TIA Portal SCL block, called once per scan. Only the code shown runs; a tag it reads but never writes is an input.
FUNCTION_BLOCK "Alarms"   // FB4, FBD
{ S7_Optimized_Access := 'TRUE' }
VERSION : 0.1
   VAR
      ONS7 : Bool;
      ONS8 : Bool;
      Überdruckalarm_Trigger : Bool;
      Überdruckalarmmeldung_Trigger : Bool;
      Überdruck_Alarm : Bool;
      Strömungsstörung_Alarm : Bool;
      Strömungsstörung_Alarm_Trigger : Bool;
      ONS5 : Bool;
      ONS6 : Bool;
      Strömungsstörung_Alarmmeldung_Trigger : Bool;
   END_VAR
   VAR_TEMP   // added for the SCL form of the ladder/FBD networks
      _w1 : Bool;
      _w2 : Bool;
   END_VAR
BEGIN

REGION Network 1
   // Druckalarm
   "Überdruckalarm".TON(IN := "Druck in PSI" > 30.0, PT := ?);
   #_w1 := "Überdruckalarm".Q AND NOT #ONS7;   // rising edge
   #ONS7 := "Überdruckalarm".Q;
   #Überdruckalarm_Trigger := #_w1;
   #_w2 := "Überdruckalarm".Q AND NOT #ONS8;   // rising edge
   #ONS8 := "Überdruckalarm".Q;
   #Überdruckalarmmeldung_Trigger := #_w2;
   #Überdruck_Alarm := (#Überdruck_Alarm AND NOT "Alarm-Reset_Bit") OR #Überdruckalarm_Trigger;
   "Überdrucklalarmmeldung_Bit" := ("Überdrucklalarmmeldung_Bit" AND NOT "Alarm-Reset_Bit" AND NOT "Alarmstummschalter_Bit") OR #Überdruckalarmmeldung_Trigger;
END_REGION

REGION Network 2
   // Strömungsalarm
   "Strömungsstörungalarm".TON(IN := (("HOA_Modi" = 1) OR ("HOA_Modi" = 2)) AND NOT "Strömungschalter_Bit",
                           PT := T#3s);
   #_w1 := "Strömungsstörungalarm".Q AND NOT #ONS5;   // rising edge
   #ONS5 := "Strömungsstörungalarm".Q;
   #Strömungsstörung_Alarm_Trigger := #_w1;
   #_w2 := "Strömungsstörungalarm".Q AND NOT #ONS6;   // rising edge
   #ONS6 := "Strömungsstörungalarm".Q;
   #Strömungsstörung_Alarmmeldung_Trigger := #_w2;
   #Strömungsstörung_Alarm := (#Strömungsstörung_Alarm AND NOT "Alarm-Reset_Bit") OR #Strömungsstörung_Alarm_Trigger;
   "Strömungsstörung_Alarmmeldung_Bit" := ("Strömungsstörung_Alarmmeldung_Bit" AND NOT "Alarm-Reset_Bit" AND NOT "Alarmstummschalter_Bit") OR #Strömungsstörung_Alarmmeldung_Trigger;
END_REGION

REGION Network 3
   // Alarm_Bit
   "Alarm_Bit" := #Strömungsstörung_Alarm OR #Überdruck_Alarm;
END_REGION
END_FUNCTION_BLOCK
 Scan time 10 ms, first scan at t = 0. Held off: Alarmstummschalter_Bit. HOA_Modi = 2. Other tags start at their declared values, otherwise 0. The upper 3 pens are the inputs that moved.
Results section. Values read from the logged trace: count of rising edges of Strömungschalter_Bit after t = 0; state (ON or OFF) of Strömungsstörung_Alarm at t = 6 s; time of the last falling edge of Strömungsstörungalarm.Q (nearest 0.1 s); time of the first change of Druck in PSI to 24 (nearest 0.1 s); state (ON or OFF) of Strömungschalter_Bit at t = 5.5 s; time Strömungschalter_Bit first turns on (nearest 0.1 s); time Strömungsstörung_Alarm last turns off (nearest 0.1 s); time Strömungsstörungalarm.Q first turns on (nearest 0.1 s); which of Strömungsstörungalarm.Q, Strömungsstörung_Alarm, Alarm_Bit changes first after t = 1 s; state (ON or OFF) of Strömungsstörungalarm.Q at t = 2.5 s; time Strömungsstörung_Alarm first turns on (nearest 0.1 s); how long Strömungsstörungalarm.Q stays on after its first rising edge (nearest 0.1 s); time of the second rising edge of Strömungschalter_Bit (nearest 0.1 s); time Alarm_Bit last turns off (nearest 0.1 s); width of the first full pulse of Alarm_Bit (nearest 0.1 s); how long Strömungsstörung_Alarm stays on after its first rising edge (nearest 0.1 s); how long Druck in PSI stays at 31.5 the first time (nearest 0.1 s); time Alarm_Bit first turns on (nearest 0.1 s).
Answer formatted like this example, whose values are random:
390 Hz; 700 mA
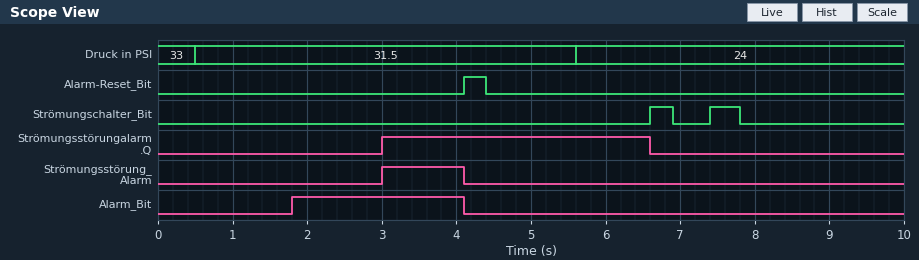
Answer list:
2; OFF; 6.6 s; 5.6 s; OFF; 6.6 s; 4.1 s; 3.0 s; Alarm_Bit; OFF; 3.0 s; 3.6 s; 7.4 s; 4.1 s; 2.3 s; 1.1 s; 5.1 s; 1.8 s
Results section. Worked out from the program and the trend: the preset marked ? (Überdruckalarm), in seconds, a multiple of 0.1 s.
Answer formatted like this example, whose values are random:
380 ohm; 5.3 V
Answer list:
1.8 s
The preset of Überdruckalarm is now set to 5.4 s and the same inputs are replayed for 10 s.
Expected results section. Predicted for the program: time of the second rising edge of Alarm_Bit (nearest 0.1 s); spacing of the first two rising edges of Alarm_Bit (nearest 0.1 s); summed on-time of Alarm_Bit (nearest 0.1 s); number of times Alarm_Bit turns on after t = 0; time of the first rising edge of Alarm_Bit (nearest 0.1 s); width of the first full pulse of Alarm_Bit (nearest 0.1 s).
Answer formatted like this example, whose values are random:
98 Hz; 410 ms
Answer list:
5.4 s; 2.4 s; 5.7 s; 2; 3.0 s; 1.1 s
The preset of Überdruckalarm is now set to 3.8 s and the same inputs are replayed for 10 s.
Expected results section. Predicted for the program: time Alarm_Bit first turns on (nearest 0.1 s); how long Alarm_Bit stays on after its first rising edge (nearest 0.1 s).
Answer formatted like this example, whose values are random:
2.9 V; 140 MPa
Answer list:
3.0 s; 1.1 s
